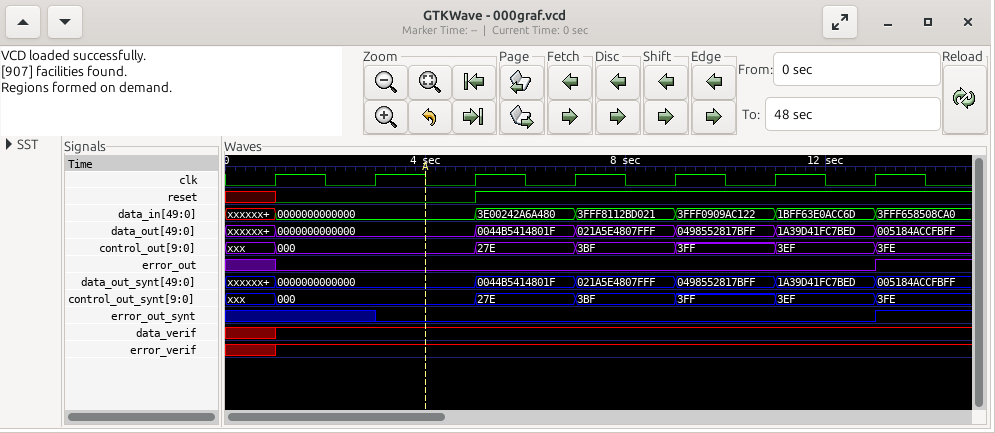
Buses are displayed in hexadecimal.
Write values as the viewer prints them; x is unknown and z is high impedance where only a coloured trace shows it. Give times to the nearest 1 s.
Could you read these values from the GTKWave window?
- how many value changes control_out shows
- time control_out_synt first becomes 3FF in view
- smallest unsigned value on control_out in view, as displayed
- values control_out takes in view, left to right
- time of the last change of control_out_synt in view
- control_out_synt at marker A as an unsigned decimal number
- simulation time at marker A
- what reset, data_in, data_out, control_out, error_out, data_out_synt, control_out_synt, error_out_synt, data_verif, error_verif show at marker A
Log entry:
6
9 s
000
xxx, 000, 27E, 3BF, 3FF, 3EF, 3FE
13 s
0
4 s
reset=0, data_in=0000000000000, data_out=0000000000000, control_out=000, error_out=0, data_out_synt=0000000000000, control_out_synt=000, error_out_synt=0, data_verif=1, error_verif=1
